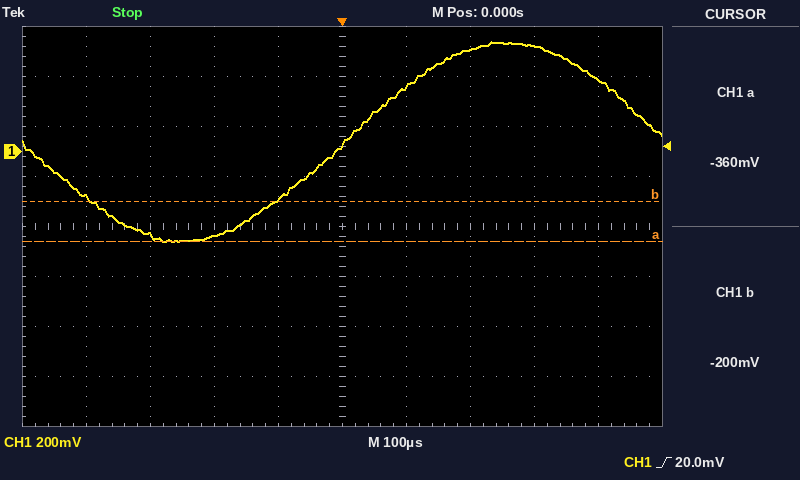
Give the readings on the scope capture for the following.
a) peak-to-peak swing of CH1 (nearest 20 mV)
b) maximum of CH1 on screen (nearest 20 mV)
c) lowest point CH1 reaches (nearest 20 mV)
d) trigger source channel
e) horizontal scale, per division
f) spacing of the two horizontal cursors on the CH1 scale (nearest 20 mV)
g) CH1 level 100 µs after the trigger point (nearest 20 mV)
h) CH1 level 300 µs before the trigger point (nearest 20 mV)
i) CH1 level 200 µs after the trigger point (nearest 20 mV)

800 mV
440 mV
-360 mV
CH1
100 µs
160 mV
260 mV
-340 mV
400 mV
